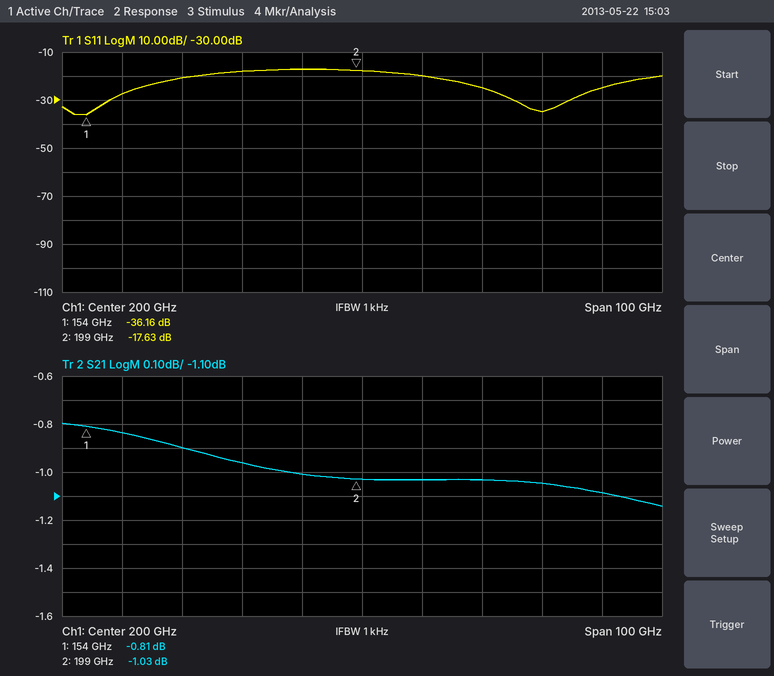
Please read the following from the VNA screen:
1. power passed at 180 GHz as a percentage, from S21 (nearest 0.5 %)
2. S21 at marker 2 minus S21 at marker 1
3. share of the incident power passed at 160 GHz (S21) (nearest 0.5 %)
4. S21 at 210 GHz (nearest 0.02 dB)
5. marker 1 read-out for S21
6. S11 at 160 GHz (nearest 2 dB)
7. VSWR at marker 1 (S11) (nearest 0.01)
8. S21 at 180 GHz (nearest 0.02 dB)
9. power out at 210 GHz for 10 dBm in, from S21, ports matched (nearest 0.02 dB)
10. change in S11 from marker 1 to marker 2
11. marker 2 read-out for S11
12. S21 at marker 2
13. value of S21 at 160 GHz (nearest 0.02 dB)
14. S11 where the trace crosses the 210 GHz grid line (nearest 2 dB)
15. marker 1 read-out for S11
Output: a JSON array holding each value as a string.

["80.0 %", "-0.22 dB", "82.5 %", "-1.04 dB", "-0.81 dB", "-28 dB", "1.03", "-0.96 dB", "8.96 dBm", "18.53 dB", "-17.63 dB", "-1.03 dB", "-0.84 dB", "-20 dB", "-36.16 dB"]
